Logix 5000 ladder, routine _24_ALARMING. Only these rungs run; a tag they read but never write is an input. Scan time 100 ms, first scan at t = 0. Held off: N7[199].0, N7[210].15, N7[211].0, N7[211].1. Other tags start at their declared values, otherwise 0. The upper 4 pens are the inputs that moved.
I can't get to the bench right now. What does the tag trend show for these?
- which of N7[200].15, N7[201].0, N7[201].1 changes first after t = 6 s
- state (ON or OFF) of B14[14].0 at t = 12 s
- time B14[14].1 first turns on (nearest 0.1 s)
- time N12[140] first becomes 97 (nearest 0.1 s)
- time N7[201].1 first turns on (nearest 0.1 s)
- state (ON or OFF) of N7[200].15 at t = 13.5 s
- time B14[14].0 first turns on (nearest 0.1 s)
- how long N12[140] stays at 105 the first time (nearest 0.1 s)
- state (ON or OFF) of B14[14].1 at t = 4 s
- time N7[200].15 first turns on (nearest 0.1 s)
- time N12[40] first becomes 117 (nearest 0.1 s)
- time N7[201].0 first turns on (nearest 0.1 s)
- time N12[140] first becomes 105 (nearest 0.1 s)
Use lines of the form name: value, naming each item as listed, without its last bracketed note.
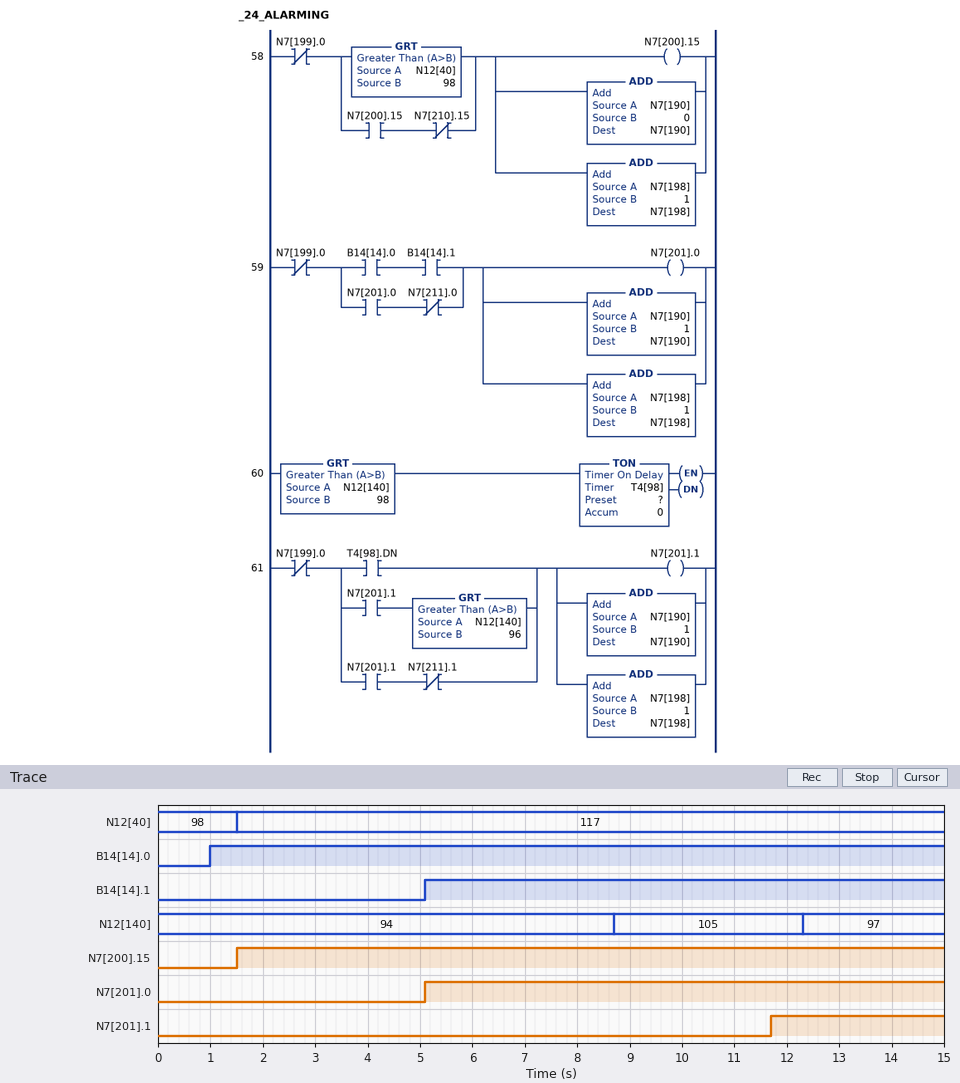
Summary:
which of N7[200].15, N7[201].0, N7[201].1 changes first after t = 6 s: N7[201].1
state (ON or OFF) of B14[14].0 at t = 12 s: ON
time B14[14].1 first turns on: 5.1 s
time N12[140] first becomes 97: 12.3 s
time N7[201].1 first turns on: 11.7 s
state (ON or OFF) of N7[200].15 at t = 13.5 s: ON
time B14[14].0 first turns on: 1.0 s
how long N12[140] stays at 105 the first time: 3.6 s
state (ON or OFF) of B14[14].1 at t = 4 s: OFF
time N7[200].15 first turns on: 1.5 s
time N12[40] first becomes 117: 1.5 s
time N7[201].0 first turns on: 5.1 s
time N12[140] first becomes 105: 8.7 s
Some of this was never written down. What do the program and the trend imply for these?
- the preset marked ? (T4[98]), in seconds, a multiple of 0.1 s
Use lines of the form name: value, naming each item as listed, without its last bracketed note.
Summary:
the preset marked ? (T4[98]), in seconds, a multiple of 0.1 s: 3.0 s
